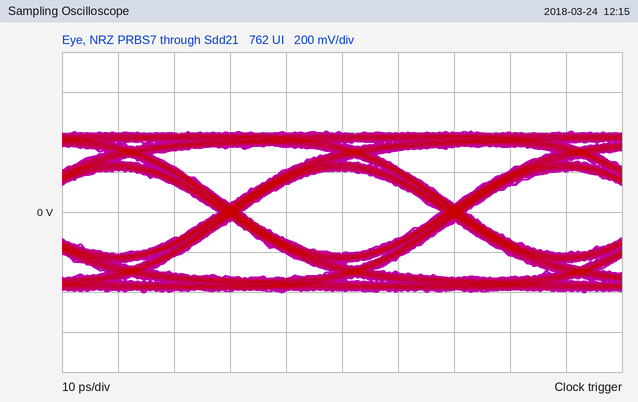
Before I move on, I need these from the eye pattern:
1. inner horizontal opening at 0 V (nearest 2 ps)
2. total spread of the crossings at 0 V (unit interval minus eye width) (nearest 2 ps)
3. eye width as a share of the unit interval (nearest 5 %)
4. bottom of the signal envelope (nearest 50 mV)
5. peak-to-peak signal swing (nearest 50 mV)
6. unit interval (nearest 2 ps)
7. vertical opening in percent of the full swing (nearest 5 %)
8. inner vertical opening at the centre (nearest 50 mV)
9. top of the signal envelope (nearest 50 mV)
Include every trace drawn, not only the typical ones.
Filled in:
36 ps
4 ps
90 %
-400 mV
800 mV
40 ps
50 %
400 mV
400 mV
